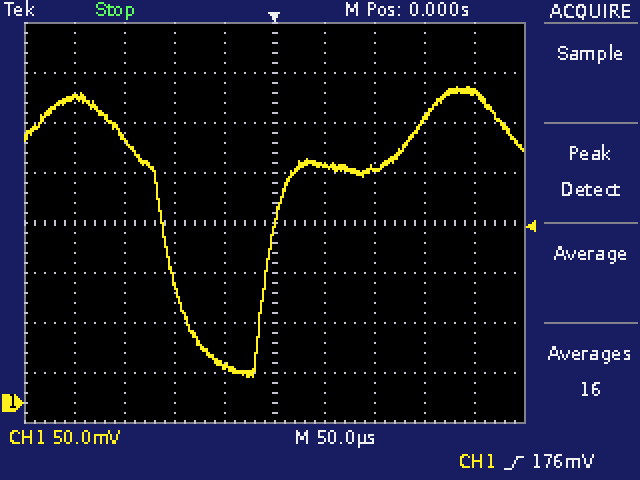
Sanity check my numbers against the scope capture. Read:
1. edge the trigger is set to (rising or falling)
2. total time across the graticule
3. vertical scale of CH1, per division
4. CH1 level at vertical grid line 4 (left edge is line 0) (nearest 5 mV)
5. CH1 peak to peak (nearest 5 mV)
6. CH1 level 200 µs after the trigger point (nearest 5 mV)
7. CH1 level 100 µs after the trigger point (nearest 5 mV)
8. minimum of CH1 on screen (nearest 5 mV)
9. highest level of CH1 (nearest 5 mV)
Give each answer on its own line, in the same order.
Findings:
rising
500 µs
50 mV
40 mV
290 mV
310 mV
235 mV
25 mV
315 mV
